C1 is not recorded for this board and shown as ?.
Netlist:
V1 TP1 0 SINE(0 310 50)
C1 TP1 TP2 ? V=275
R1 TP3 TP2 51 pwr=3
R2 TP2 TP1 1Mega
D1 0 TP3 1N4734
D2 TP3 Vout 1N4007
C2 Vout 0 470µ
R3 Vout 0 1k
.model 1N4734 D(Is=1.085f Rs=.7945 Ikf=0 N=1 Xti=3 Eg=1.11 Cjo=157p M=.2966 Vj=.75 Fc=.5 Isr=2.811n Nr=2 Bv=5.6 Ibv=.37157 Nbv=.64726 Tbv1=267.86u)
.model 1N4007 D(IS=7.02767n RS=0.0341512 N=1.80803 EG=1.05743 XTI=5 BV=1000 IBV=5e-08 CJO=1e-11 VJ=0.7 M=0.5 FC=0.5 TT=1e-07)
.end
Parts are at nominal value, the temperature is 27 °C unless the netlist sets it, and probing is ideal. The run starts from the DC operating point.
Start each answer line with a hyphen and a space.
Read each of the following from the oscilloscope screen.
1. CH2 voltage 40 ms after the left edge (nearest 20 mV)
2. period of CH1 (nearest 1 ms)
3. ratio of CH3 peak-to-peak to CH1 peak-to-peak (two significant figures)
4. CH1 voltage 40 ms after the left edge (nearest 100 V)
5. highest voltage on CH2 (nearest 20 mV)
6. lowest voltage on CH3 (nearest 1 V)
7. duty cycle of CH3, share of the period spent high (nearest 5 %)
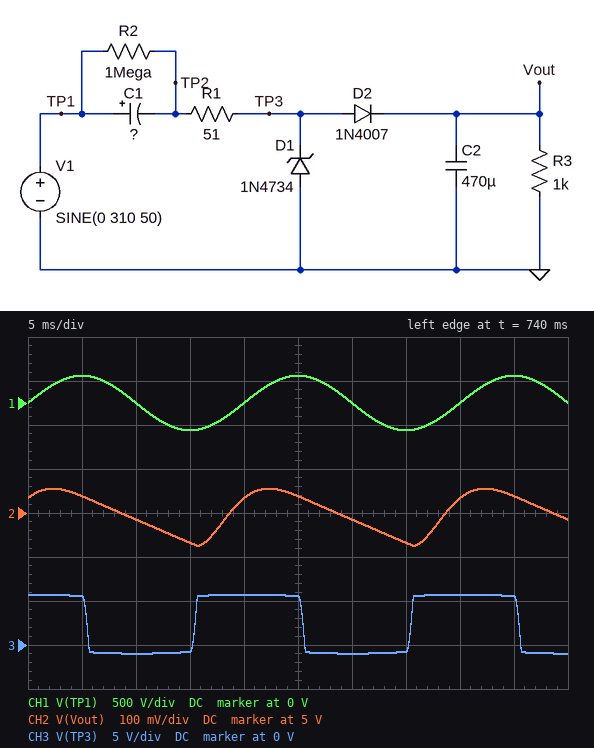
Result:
- 5.04 V
- 20 ms
- 0.011
- 0 V
- 5.06 V
- -1 V
- 50 %
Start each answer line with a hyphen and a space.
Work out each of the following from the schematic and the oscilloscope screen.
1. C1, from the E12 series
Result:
- 1.8 µF
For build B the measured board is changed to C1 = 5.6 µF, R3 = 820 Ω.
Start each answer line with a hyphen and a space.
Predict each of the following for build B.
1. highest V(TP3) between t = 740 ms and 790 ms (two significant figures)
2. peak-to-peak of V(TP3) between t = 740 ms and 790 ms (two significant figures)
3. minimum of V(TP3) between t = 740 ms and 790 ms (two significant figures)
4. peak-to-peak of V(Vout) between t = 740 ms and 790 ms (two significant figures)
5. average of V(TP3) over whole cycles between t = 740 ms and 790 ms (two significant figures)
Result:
- 6.0 V
- 7.3 V
- -1.3 V
- 190 mV
- 2.4 V
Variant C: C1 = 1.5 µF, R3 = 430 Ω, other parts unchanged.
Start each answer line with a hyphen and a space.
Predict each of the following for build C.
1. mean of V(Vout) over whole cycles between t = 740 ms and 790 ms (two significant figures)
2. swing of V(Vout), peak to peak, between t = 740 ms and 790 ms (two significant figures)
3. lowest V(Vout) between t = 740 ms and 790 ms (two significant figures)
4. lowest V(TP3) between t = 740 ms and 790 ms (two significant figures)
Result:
- 4.9 V
- 290 mV
- 4.7 V
- -950 mV
